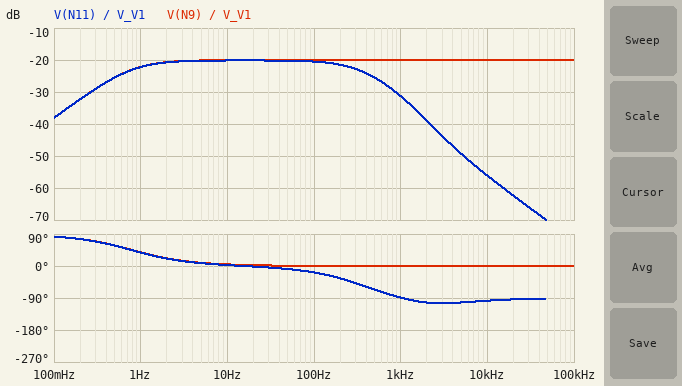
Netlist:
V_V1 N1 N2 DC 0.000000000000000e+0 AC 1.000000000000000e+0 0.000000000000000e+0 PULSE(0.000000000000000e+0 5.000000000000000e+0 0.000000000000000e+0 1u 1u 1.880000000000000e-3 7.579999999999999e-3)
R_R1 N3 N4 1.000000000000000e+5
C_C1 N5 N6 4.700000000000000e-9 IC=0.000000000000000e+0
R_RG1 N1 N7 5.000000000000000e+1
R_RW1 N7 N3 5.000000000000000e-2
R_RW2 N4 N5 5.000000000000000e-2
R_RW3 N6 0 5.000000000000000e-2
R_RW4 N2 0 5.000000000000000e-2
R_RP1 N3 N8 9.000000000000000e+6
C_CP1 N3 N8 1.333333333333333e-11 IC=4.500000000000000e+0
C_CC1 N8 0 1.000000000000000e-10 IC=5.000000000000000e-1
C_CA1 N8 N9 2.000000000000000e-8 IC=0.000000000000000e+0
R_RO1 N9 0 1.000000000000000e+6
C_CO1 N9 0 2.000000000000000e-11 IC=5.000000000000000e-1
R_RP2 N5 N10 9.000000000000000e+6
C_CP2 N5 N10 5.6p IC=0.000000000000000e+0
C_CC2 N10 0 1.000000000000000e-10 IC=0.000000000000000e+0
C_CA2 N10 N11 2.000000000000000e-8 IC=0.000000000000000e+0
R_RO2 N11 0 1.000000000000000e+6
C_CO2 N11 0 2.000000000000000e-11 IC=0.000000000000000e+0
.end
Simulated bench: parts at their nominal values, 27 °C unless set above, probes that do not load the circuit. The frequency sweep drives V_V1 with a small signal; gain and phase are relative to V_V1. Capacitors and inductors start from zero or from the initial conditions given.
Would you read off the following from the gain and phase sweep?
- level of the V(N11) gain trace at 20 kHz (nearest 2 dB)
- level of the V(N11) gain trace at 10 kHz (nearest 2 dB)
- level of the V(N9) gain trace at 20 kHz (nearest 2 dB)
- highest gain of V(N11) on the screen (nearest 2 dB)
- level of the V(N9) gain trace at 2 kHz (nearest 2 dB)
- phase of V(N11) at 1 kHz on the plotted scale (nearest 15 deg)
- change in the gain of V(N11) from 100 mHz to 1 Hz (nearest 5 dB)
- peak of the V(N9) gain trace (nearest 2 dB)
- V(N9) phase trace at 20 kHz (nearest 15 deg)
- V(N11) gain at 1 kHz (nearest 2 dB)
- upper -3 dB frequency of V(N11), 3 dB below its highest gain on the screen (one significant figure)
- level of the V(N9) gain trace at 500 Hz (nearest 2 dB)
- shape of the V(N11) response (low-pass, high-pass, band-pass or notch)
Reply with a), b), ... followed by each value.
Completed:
a) -62 dB
b) -56 dB
c) -20 dB
d) -20 dB
e) -20 dB
f) -90 deg
g) 15 dB
h) -20 dB
i) 0 deg
j) -32 dB
k) 300 Hz
l) -20 dB
m) band-pass
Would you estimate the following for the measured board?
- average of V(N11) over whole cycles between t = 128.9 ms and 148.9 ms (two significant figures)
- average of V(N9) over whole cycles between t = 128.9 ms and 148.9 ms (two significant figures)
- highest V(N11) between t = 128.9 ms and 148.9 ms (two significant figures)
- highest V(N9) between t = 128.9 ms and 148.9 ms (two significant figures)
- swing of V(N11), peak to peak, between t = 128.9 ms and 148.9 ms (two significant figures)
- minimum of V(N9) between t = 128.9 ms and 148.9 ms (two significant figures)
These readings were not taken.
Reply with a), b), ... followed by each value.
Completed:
a) 62 mV
b) 62 mV
c) 420 mV
d) 440 mV
e) 490 mV
f) -68 mV
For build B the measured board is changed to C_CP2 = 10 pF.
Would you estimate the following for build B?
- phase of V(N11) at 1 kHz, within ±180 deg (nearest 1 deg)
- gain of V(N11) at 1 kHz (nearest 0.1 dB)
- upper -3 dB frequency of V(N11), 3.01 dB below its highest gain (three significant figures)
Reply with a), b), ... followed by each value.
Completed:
a) -78 deg
b) -30.6 dB
c) 335 Hz
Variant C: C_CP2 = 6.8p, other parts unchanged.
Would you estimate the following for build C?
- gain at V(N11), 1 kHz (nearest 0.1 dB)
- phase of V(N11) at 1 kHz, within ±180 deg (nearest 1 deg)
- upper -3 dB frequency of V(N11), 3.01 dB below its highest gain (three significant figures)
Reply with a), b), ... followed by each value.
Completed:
a) -31.1 dB
b) -86 deg
c) 330 Hz
